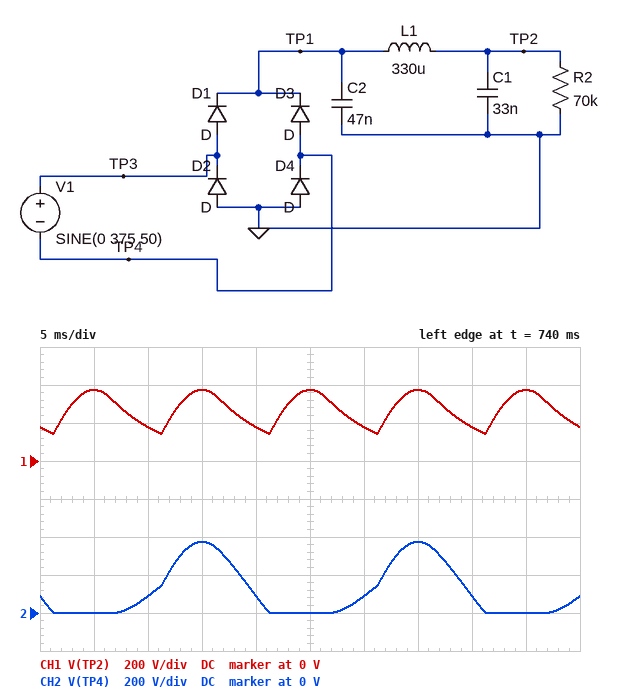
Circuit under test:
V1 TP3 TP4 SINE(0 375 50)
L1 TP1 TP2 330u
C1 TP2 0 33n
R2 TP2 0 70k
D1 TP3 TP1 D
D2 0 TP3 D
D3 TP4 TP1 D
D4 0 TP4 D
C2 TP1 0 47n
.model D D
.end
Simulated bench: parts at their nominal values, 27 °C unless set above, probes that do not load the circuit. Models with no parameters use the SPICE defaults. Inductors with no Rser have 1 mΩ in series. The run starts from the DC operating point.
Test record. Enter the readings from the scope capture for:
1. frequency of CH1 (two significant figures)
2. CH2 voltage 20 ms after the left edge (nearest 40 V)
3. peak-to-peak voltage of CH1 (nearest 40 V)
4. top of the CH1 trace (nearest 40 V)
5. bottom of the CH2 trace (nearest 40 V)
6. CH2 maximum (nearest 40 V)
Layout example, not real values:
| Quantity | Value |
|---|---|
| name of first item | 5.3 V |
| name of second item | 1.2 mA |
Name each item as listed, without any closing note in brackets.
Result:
| Quantity | Value |
|---|---|
| frequency of CH1 | 100 Hz |
| CH2 voltage 20 ms after the left edge | 80 V |
| peak-to-peak voltage of CH1 | 240 V |
| top of the CH1 trace | 360 V |
| bottom of the CH2 trace | 0 V |
| CH2 maximum | 360 V |
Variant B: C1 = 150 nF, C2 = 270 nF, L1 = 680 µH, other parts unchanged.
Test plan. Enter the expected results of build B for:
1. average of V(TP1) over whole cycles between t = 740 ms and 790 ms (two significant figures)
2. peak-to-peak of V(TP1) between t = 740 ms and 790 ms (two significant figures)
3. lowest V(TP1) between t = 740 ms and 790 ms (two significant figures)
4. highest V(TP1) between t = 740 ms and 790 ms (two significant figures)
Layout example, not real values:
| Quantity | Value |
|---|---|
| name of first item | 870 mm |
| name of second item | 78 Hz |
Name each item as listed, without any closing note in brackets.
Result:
| Quantity | Value |
|---|---|
| average of V(TP1) over whole cycles between t = 740 ms and 790 ms | 330 V |
| peak-to-peak of V(TP1) between t = 740 ms and 790 ms | 85 V |
| lowest V(TP1) between t = 740 ms and 790 ms | 290 V |
| highest V(TP1) between t = 740 ms and 790 ms | 370 V |
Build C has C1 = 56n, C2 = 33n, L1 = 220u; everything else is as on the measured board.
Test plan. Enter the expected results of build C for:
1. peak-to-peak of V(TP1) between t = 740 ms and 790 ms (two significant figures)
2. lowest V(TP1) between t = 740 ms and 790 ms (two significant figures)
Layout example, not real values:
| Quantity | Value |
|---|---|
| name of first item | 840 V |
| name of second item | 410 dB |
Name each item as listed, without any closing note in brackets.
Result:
| Quantity | Value |
|---|---|
| peak-to-peak of V(TP1) between t = 740 ms and 790 ms | 220 V |
| lowest V(TP1) between t = 740 ms and 790 ms | 150 V |
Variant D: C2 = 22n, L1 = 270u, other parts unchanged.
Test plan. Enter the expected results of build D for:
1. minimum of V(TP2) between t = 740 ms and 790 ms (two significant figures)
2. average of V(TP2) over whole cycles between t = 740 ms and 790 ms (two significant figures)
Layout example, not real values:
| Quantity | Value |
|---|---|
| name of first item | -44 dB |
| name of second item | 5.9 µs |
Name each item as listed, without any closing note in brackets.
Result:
| Quantity | Value |
|---|---|
| minimum of V(TP2) between t = 740 ms and 790 ms | 110 V |
| average of V(TP2) over whole cycles between t = 740 ms and 790 ms | 260 V |
